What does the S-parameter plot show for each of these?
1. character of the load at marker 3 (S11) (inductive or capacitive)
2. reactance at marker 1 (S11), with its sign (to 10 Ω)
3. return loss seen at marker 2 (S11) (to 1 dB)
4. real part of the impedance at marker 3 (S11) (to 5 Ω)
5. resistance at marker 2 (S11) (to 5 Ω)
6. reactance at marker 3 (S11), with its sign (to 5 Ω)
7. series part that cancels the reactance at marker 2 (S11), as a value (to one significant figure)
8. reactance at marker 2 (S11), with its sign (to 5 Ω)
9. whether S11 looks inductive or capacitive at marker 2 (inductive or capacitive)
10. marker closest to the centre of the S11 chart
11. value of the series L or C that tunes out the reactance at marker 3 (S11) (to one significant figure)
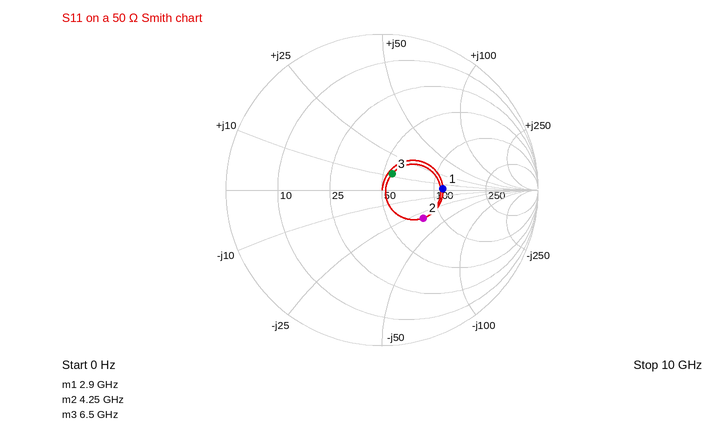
inductive
0 Ω
10 dB
55 Ω
80 Ω
+10 Ω
1 nH
-30 Ω
capacitive
marker 3
2 pF
